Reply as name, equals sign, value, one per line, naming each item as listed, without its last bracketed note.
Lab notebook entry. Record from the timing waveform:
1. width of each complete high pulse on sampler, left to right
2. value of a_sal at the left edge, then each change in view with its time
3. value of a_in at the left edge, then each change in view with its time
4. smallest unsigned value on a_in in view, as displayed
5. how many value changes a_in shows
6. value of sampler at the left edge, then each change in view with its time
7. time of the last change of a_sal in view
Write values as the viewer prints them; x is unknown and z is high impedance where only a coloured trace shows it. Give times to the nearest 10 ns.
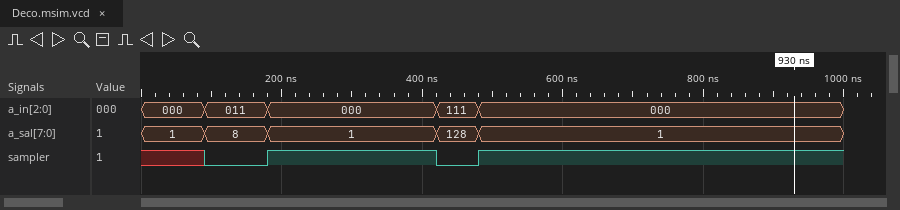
width of each complete high pulse on sampler, left to right = 240 ns
value of a_sal at the left edge, then each change in view with its time = 1, 8 at 90 ns, 1 at 180 ns, 128 at 420 ns, 1 at 480 ns
value of a_in at the left edge, then each change in view with its time = 000, 011 at 90 ns, 000 at 180 ns, 111 at 420 ns, 000 at 480 ns
smallest unsigned value on a_in in view, as displayed = 000
how many value changes a_in shows = 4
value of sampler at the left edge, then each change in view with its time = x, 0 at 90 ns, 1 at 180 ns, 0 at 420 ns, 1 at 480 ns
time of the last change of a_sal in view = 480 ns
